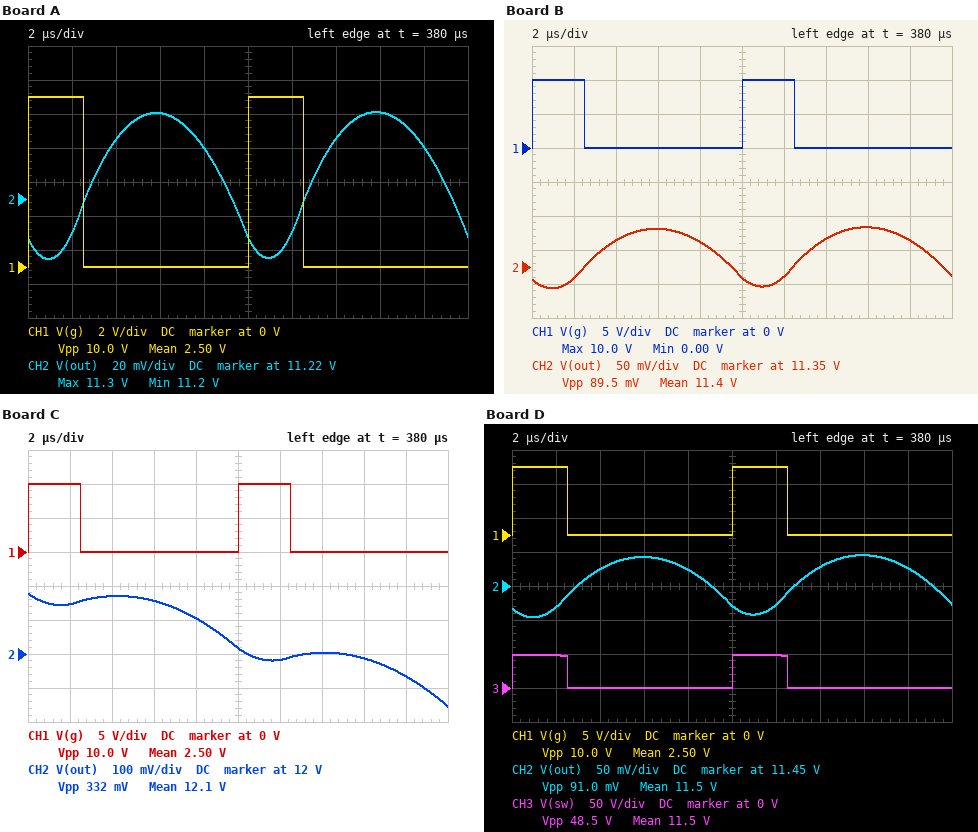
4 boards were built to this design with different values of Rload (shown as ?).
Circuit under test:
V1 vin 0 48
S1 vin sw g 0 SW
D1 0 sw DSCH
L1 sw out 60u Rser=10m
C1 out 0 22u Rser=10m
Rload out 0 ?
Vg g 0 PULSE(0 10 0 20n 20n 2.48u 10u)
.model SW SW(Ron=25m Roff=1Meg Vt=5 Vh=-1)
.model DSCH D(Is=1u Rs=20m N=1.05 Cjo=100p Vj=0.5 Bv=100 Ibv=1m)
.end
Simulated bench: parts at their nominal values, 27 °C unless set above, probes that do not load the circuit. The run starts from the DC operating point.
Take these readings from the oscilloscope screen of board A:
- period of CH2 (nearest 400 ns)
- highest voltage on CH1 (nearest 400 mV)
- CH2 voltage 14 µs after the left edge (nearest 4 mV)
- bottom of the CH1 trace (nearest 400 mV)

10.0 µs
10.0 V
11.256 V
0 V
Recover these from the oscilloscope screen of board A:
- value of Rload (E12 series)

0.82 Ω
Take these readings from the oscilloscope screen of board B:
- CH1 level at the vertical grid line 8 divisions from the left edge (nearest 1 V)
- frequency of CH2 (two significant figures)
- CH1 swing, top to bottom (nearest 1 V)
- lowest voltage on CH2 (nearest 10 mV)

0 V
100 kHz
10 V
11.32 V
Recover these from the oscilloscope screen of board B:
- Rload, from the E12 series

1.2 Ω
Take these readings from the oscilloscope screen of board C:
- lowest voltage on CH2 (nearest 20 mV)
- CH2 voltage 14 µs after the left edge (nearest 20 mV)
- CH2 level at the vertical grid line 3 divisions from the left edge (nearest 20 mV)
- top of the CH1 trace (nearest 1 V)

11.84 V
12.00 V
12.16 V
10 V
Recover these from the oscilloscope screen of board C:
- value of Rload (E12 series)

3.3 Ω
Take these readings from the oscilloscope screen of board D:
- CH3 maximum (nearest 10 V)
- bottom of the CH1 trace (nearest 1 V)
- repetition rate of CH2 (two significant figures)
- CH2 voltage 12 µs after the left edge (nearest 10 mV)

50 V
0 V
100 kHz
11.42 V
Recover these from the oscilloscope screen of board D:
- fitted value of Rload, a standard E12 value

1.5 Ω
